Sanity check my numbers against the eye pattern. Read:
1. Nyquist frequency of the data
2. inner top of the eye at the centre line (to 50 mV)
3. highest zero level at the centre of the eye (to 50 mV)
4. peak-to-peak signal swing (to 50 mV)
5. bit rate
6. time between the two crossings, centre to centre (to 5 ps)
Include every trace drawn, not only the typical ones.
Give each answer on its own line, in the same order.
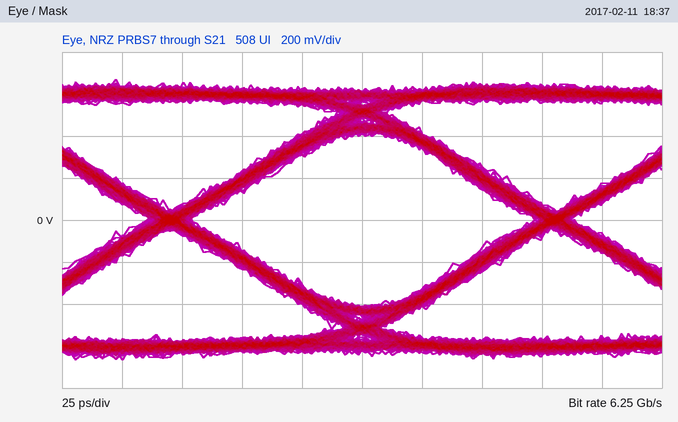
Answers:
3.125 GHz
400 mV
-400 mV
1.35 V
6.25 Gb/s
160 ps
